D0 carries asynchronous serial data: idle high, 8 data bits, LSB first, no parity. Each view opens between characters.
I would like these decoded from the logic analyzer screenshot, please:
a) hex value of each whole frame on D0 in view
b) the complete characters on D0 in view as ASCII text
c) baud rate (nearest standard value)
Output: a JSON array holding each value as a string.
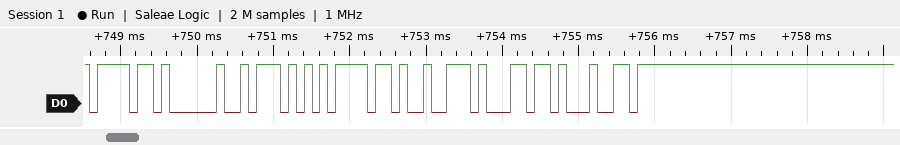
["6F, 20, 57, 6F, 72, 6C, 64", "\"o World\"", "9600 baud"]
